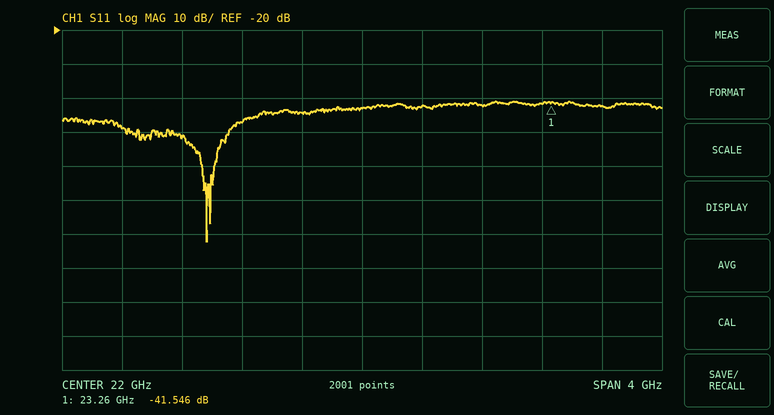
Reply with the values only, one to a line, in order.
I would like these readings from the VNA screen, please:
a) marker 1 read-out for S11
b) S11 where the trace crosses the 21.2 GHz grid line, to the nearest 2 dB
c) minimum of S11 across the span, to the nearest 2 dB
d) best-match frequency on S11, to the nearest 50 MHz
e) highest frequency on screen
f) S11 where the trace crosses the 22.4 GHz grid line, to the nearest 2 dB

-41.546 dB
-48 dB
-82 dB
20.95 GHz
24 GHz
-42 dB
